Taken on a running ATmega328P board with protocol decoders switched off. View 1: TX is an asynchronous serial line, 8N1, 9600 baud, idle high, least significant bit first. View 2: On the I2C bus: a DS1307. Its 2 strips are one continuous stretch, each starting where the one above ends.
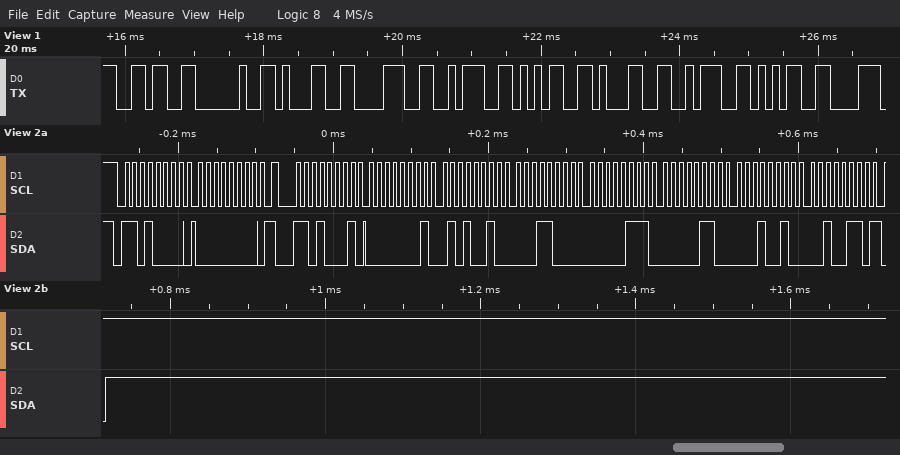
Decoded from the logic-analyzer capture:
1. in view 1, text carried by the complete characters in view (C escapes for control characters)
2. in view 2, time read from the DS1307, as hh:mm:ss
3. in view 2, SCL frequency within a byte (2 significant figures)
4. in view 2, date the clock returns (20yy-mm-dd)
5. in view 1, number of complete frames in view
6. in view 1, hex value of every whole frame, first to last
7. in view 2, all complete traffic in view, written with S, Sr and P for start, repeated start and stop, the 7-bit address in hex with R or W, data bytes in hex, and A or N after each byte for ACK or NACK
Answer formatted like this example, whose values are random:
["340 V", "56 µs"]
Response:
["\"6 18:51:5\"", "18:52:01", "100 kHz", "2026-12-06", "9", "36 20 31 38 3A 35 31 3A 35", "S 68W A 00 A Sr 68R A 01 A 52 A 18 A 07 A 06 A 12 A 26 N P"]
